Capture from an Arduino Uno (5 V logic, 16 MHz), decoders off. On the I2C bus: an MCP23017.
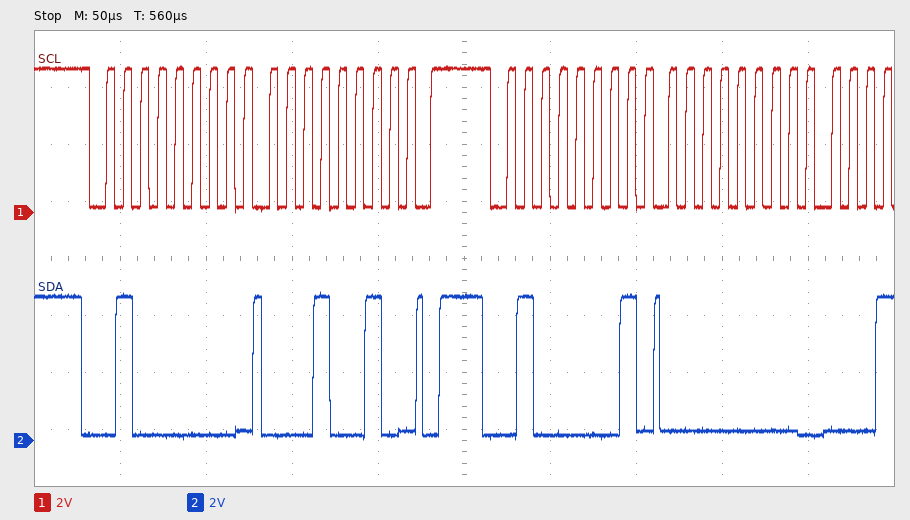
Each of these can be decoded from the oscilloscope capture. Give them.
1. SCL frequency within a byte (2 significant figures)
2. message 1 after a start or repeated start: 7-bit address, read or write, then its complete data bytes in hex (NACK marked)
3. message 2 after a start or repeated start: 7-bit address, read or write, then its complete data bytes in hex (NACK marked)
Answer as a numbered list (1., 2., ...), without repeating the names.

1. 100 kHz
2. 0x20 write: 12
3. 0x20 read: 00
